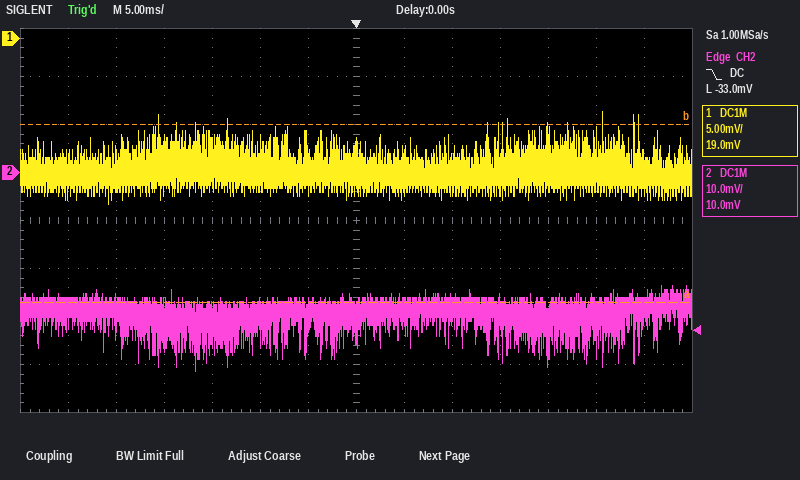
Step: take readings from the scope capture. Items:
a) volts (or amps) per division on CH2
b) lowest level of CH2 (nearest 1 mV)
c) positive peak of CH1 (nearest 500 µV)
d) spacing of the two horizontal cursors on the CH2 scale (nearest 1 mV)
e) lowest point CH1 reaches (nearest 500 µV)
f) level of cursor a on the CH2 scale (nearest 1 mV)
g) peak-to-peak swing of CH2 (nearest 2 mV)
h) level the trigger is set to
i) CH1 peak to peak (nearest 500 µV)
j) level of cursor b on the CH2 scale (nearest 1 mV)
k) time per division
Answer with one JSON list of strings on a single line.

["10 mV", "-41 mV", "-7.5 mV", "37 mV", "-17.0 mV", "-27 mV", "18 mV", "-33.0 mV", "9.5 mV", "10 mV", "5 ms"]
